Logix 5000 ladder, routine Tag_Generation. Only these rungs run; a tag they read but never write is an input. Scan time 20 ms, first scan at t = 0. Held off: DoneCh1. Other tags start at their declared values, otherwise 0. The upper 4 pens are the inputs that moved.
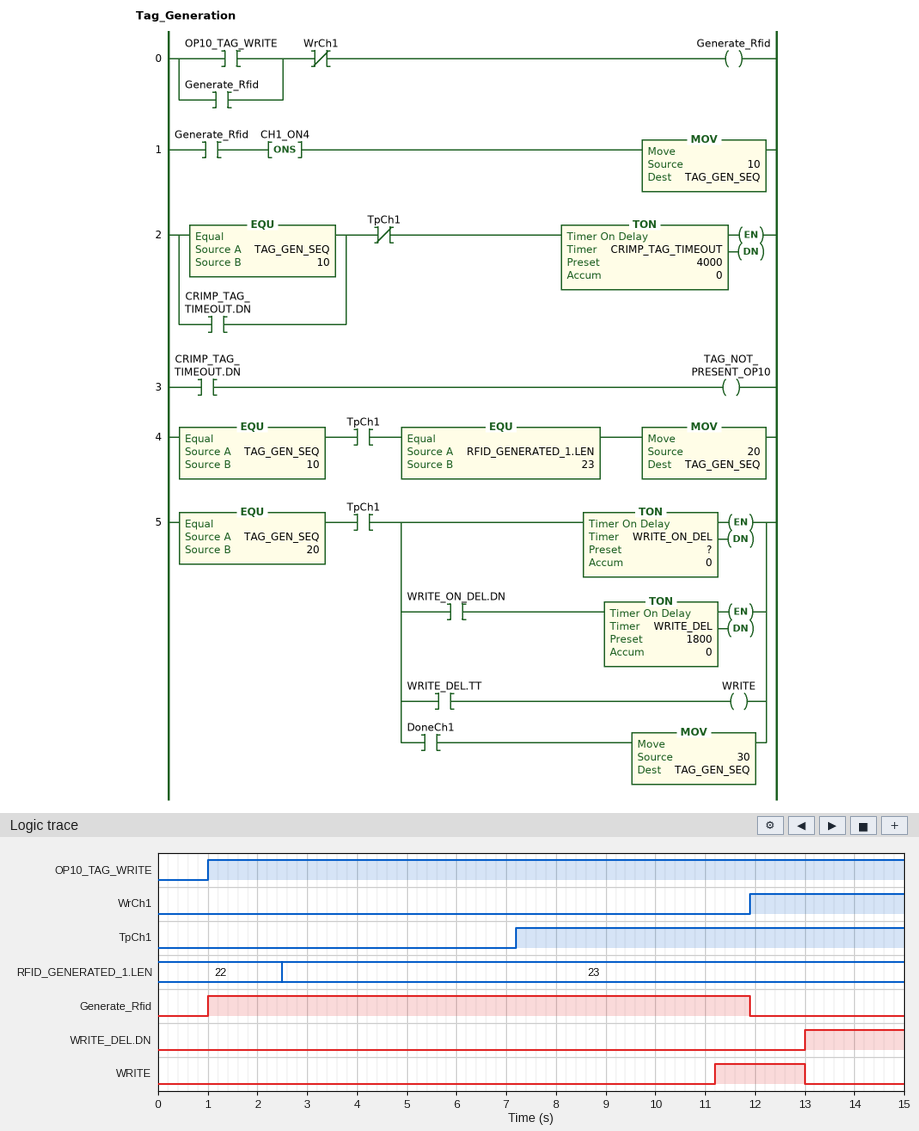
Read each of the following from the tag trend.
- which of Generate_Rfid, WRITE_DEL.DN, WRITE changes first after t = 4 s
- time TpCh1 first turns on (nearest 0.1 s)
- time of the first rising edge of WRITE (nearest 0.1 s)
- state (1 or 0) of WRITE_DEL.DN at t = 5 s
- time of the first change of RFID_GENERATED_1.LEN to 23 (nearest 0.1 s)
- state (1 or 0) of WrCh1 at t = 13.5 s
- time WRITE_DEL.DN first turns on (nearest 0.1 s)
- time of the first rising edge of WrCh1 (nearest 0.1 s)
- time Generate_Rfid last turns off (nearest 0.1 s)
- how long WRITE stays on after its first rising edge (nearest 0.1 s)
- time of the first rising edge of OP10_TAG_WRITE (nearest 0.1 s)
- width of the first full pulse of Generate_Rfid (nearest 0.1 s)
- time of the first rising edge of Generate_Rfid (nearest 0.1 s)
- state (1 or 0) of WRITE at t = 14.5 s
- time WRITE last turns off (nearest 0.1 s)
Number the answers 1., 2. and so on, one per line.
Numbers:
1. WRITE
2. 7.2 s
3. 11.2 s
4. 0
5. 2.5 s
6. 1
7. 13.0 s
8. 11.9 s
9. 11.9 s
10. 1.8 s
11. 1.0 s
12. 10.9 s
13. 1.0 s
14. 0
15. 13.0 s
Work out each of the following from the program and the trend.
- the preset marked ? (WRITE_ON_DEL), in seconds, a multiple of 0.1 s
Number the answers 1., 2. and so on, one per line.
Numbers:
1. 4.0 s
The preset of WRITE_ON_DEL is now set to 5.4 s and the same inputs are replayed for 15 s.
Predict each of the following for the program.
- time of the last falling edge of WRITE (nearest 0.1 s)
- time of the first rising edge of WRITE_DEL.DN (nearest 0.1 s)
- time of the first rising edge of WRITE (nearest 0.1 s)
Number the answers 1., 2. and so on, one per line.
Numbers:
1. 14.4 s
2. 14.4 s
3. 12.6 s
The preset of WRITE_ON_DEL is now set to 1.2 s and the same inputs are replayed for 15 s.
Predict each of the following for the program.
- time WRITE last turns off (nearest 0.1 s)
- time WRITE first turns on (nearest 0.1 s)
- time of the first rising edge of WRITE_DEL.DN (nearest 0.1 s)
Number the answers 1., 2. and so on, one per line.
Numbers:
1. 10.2 s
2. 8.4 s
3. 10.2 s
